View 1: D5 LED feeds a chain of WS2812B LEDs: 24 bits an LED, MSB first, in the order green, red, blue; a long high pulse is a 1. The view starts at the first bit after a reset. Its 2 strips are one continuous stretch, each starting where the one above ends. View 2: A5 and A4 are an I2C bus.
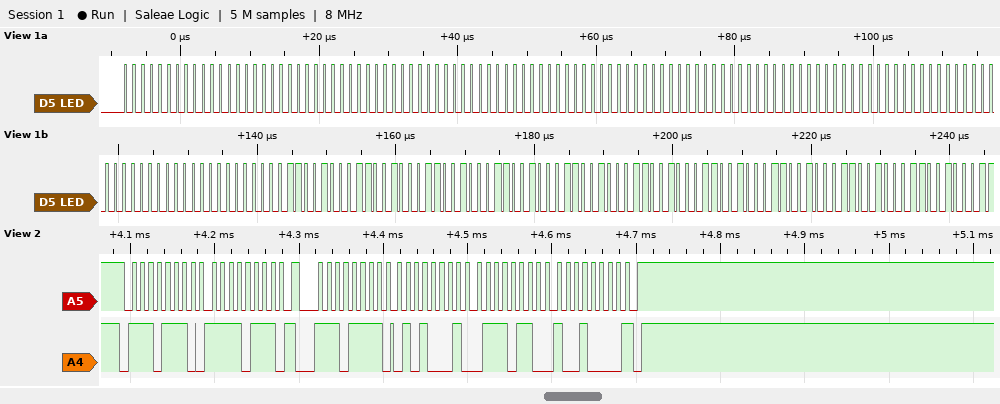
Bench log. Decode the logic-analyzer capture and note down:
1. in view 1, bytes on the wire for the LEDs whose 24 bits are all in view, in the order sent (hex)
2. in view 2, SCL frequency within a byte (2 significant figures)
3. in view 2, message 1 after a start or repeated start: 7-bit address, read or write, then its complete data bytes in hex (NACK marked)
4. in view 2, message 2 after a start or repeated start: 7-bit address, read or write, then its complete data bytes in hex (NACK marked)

00 00 00 00 00 00 00 00 00 00 00 00 00 00 00 32 32 32 32 32 32 32 32 32
100 kHz
0x77 write: F7
0x77 read: 51 76 90 NACK
